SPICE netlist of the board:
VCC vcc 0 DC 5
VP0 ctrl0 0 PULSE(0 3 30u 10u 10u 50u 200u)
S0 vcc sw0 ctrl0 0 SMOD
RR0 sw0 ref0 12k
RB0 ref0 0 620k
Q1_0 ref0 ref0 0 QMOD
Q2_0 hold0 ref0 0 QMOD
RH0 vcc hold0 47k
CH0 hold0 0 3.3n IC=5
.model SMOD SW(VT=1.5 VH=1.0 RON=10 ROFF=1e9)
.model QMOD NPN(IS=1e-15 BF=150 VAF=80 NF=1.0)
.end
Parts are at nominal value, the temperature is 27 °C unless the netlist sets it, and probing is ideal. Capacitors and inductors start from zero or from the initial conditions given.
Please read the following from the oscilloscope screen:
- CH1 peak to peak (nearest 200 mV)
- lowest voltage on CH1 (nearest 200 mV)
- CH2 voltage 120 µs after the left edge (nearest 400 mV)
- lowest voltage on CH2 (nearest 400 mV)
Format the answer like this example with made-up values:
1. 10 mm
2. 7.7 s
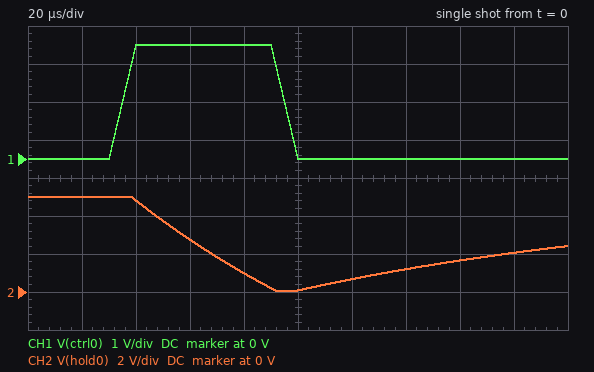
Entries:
1. 3.0 V
2. 0 V
3. 800 mV
4. 0 V
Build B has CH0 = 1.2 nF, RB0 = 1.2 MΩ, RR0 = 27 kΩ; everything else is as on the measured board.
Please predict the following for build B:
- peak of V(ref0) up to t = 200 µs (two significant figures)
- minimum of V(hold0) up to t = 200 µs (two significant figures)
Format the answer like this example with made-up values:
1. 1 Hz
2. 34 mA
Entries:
1. 670 mV
2. 92 mV
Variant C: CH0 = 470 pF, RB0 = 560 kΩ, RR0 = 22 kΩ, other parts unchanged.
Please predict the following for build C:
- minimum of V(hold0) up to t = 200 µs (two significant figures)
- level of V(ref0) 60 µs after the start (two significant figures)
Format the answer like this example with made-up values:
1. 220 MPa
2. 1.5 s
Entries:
1. 45 mV
2. 670 mV
